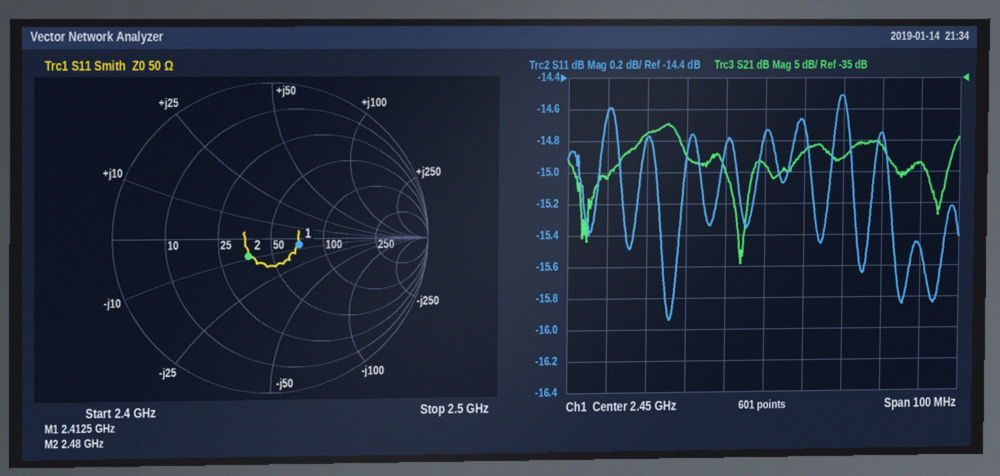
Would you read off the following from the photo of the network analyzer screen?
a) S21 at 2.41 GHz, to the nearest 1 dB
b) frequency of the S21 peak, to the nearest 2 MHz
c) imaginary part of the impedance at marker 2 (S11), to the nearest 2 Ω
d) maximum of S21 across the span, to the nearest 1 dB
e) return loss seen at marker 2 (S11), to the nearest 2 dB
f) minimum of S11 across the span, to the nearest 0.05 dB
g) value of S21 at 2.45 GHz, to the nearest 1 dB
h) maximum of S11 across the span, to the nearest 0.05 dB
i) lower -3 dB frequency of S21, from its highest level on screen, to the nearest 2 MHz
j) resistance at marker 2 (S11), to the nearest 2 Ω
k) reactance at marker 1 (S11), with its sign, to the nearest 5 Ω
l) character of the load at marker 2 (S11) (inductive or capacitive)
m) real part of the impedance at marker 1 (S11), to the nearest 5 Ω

-51 dB
2.426 GHz
-8 Ω
-42 dB
14 dB
-15.95 dB
-49 dB
-14.50 dB
2.418 GHz
36 Ω
-5 Ω
capacitive
70 Ω
